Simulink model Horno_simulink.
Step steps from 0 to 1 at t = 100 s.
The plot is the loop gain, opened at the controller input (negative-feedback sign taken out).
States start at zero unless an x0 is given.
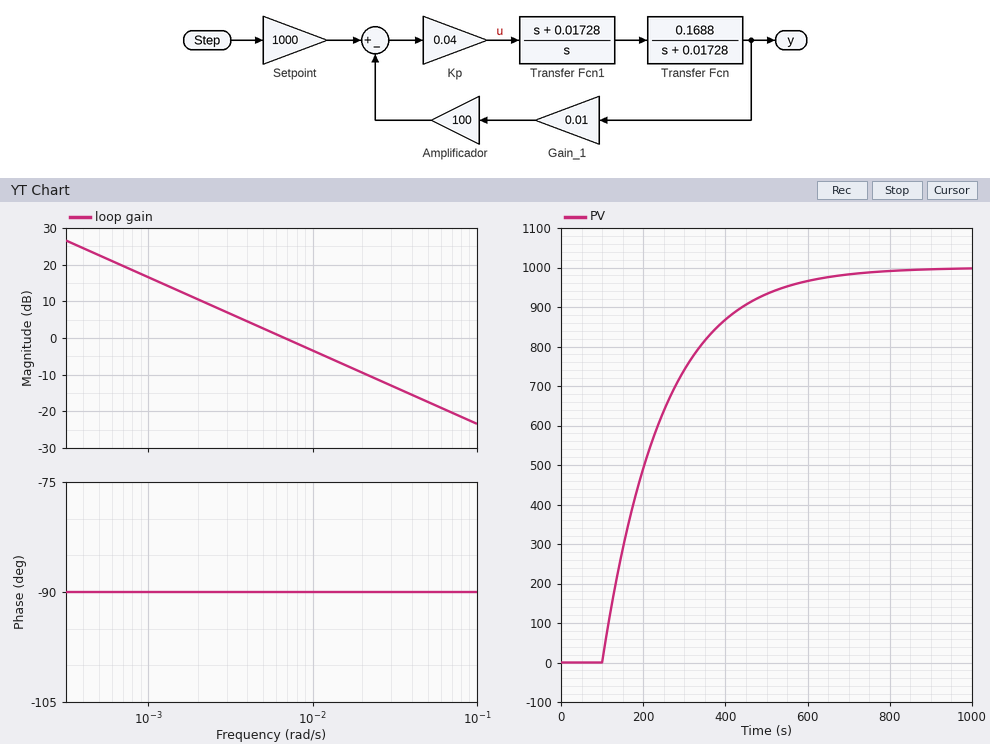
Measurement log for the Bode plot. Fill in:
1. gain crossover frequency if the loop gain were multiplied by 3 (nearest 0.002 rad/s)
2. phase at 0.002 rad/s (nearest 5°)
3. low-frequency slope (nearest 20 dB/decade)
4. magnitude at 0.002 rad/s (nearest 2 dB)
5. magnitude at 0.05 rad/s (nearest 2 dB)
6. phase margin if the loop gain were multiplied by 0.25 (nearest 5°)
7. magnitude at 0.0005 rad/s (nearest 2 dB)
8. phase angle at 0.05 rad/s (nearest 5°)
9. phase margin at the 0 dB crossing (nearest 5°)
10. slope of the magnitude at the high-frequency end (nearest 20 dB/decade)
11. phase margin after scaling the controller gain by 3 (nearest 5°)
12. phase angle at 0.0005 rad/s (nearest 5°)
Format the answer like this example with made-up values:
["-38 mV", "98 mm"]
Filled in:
["0.020 rad/s", "-90°", "-20 dB/decade", "10 dB", "-18 dB", "90°", "22 dB", "-90°", "90°", "-20 dB/decade", "90°", "-90°"]
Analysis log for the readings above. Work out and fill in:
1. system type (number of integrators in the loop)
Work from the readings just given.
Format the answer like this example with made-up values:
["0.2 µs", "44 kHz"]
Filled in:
["1"]
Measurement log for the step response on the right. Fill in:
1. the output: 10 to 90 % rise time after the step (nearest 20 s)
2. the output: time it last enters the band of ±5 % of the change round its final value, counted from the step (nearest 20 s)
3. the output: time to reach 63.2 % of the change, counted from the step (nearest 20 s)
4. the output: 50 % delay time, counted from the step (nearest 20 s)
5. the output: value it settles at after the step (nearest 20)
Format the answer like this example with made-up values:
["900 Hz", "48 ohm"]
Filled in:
["320 s", "440 s", "140 s", "100 s", "1000"]
